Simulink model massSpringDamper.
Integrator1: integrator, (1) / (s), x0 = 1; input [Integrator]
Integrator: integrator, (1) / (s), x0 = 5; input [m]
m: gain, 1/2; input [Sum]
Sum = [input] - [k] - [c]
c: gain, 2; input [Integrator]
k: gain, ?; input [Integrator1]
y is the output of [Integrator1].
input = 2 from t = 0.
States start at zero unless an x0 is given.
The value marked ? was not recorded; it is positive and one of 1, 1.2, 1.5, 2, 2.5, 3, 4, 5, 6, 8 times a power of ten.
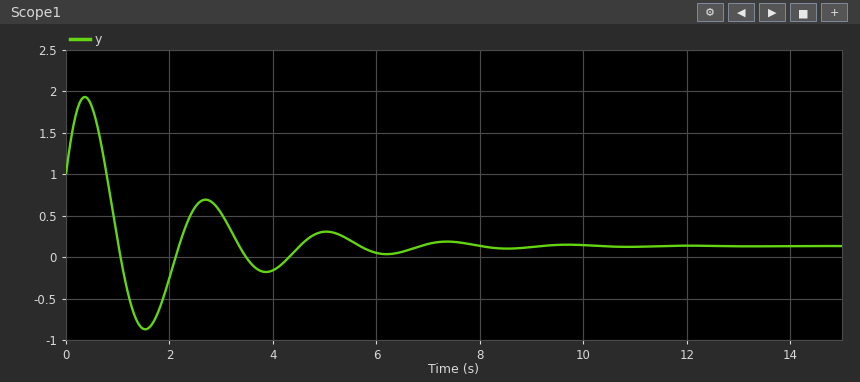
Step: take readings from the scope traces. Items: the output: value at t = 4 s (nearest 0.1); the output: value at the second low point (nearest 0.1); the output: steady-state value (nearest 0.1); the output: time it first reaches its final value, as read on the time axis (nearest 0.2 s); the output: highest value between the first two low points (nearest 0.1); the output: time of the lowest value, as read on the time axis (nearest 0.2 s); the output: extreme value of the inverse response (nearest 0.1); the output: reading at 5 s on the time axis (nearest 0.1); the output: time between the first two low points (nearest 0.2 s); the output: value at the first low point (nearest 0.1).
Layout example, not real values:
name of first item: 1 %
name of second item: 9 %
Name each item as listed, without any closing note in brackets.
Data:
the output: value at t = 4 s: -0.2
the output: value at the second low point: -0.2
the output: steady-state value: 0.1
the output: time it first reaches its final value, as read on the time axis: 1.0 s
the output: highest value between the first two low points: 0.7
the output: time of the lowest value, as read on the time axis: 1.6 s
the output: extreme value of the inverse response: 1.9
the output: reading at 5 s on the time axis: 0.3
the output: time between the first two low points: 2.4 s
the output: value at the first low point: -0.9
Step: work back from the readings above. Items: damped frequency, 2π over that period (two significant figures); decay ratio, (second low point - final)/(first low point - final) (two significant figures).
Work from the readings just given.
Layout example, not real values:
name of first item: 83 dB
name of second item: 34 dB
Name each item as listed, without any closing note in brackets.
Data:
damped frequency, 2π over that period: 2.6 rad/s
decay ratio, (second low point - final)/(first low point - final): 0.30
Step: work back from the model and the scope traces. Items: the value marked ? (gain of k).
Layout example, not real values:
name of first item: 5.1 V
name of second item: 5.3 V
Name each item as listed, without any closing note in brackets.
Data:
the value marked ?: 15
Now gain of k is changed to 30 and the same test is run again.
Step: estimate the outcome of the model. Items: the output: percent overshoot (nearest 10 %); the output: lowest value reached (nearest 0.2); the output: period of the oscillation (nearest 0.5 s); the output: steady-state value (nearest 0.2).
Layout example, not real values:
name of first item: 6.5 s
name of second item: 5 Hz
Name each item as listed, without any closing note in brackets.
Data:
the output: percent overshoot: 110 %
the output: lowest value reached: -1.0
the output: period of the oscillation: 1.5 s
the output: steady-state value: 0.0
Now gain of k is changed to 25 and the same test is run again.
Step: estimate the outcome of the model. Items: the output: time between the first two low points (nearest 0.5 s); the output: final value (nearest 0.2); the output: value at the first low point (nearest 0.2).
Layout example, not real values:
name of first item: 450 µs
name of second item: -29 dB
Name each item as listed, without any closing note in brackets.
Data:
the output: time between the first two low points: 2.0 s
the output: final value: 0.0
the output: value at the first low point: -1.0
